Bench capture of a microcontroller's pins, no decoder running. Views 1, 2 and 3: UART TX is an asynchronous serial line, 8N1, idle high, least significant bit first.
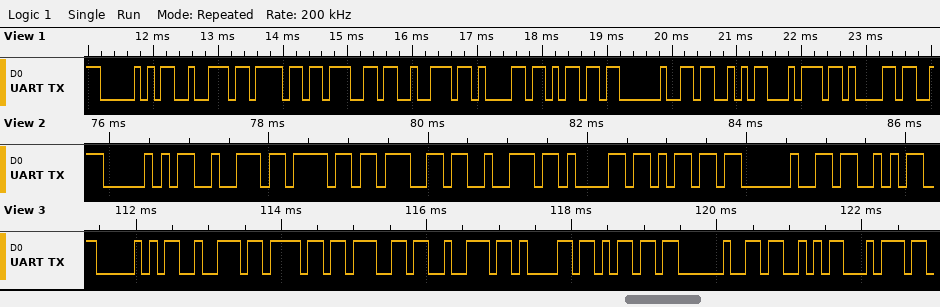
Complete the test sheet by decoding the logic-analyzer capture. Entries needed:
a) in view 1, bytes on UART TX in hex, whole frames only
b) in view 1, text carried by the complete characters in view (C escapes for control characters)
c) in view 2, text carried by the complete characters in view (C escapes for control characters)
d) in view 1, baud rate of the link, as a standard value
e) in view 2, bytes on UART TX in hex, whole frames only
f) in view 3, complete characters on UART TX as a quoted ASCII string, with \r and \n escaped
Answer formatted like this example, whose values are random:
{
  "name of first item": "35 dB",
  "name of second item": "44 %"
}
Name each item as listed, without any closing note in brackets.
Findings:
{
  "in view 1, bytes on UART TX in hex, whole frames only": "0x50 0x72 0x6F 0x67 0x72 0x61 0x6D 0x20 0x53 0x74 0x61",
  "in view 1, text carried by the complete characters in view": "\"Program Sta\"",
  "in view 2, text carried by the complete characters in view": "\"Program S\"",
  "in view 1, baud rate of the link, as a standard value": "9600 baud",
  "in view 2, bytes on UART TX in hex, whole frames only": "50 72 6F 67 72 61 6D 20 53",
  "in view 3, complete characters on UART TX as a quoted ASCII string, with \\r and \\n escaped": "\"Program St\""
}
